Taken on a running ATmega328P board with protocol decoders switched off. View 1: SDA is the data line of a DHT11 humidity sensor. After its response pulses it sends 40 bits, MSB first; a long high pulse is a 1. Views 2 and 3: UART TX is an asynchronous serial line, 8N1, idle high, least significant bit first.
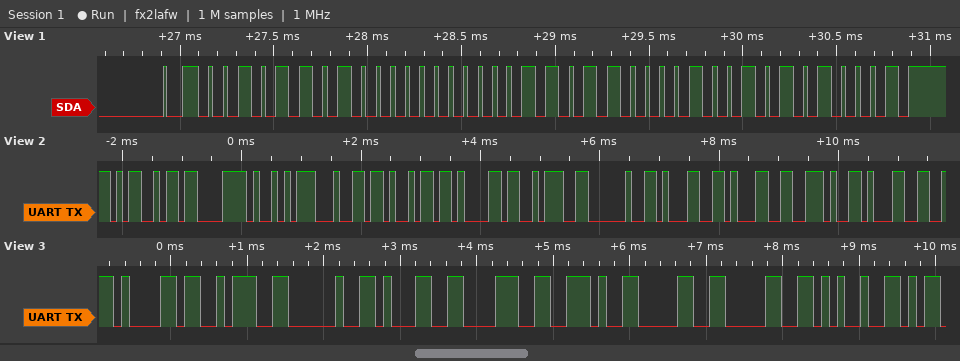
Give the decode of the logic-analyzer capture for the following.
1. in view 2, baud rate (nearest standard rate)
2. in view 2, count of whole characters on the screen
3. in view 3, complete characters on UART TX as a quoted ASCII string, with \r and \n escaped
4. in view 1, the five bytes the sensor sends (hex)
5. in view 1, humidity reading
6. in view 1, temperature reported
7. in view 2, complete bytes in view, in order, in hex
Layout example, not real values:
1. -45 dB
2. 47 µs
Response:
1. 9600 baud
2. 12
3. "a: 18.00%"
4. 2D 00 1B 09 51
5. 45 %
6. 27.9 °C
7. 4D C3 A9 64 69 61 3A 20 31 31 2E 31
